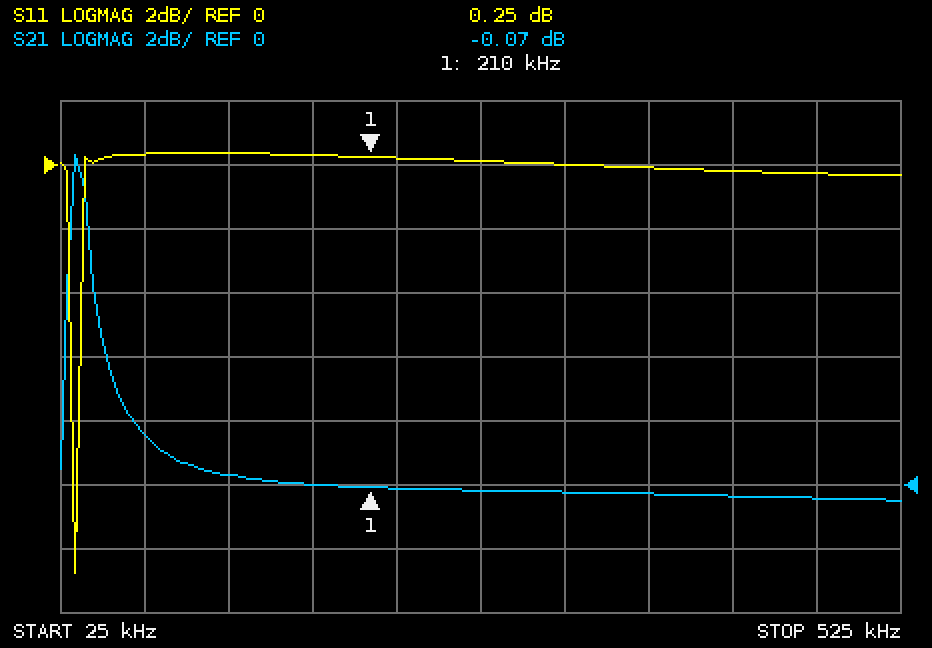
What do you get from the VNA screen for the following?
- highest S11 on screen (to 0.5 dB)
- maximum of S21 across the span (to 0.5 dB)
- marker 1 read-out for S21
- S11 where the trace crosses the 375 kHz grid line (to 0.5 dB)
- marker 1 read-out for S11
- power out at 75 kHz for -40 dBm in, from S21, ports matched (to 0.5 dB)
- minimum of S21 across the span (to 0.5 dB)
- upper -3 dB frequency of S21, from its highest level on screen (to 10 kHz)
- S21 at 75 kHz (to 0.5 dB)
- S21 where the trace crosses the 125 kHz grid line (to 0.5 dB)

0.5 dB
10.5 dB
-0.07 dB
0.0 dB
0.25 dB
-38.5 dBm
-0.5 dB
40 kHz
1.5 dB
0.5 dB
